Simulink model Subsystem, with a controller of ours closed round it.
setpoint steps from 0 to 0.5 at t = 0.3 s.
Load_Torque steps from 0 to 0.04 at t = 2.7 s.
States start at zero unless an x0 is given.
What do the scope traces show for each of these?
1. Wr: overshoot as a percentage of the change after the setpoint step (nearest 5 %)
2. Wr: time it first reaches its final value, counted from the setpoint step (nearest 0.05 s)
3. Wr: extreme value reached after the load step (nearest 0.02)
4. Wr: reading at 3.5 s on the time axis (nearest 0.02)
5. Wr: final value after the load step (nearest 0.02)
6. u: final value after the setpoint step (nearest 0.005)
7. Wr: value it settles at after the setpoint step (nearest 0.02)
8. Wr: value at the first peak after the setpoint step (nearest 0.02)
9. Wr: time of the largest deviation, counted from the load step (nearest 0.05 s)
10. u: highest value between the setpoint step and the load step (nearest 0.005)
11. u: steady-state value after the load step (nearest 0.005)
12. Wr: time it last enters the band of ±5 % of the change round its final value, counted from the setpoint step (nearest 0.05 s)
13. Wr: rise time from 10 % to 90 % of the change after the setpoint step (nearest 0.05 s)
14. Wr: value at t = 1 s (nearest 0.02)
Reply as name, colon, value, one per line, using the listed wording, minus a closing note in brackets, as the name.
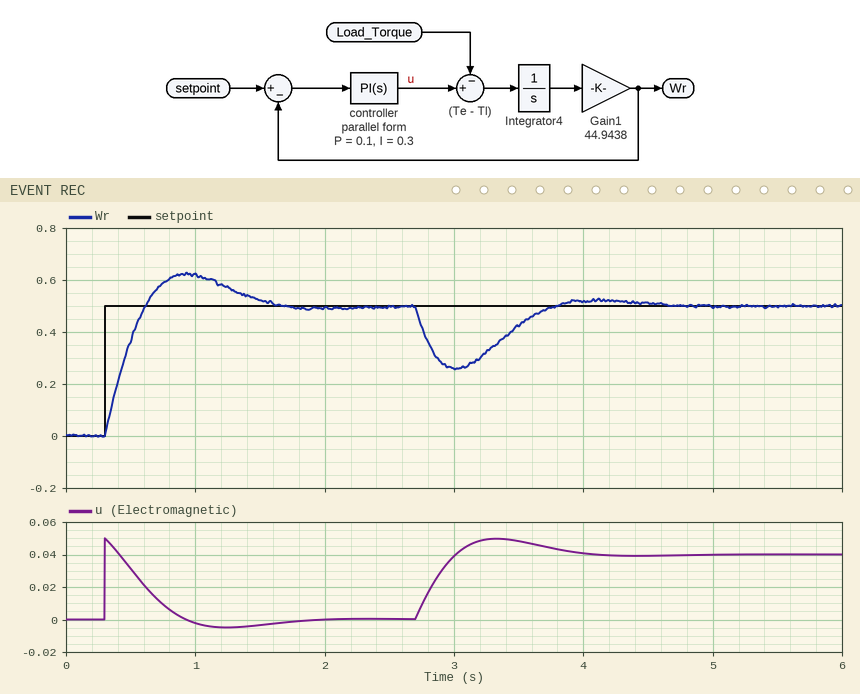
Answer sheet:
Wr: overshoot as a percentage of the change after the setpoint step: 25 %
Wr: time it first reaches its final value, counted from the setpoint step: 0.30 s
Wr: extreme value reached after the load step: 0.26
Wr: reading at 3.5 s on the time axis: 0.42
Wr: final value after the load step: 0.50
u: final value after the setpoint step: 0.000
Wr: value it settles at after the setpoint step: 0.50
Wr: value at the first peak after the setpoint step: 0.62
Wr: time of the largest deviation, counted from the load step: 0.30 s
u: highest value between the setpoint step and the load step: 0.050
u: steady-state value after the load step: 0.040
Wr: time it last enters the band of ±5 % of the change round its final value, counted from the setpoint step: 1.20 s
Wr: rise time from 10 % to 90 % of the change after the setpoint step: 0.25 s
Wr: value at t = 1 s: 0.62
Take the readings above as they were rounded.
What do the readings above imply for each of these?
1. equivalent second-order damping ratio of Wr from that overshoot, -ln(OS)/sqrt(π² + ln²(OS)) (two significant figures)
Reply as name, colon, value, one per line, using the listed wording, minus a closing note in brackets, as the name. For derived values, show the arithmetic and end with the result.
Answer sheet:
equivalent second-order damping ratio of Wr from that overshoot, -ln(OS)/sqrt(π² + ln²(OS)): ln(0.25) = -1.386; 1.386 / sqrt(9.870 + 1.922) = 0.40
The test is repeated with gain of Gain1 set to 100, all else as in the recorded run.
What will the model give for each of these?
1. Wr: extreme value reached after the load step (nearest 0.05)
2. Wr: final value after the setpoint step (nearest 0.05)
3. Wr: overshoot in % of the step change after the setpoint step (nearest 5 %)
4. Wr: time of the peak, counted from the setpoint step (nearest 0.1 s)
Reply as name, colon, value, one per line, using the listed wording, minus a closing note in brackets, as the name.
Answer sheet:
Wr: extreme value reached after the load step: 0.20
Wr: final value after the setpoint step: 0.50
Wr: overshoot in % of the step change after the setpoint step: 15 %
Wr: time of the peak, counted from the setpoint step: 0.4 s
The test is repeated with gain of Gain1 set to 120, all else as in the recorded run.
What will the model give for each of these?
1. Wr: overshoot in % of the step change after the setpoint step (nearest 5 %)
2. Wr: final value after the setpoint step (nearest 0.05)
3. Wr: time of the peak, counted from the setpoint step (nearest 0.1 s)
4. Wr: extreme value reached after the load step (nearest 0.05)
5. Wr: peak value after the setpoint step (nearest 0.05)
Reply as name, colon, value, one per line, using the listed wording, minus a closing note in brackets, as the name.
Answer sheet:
Wr: overshoot in % of the step change after the setpoint step: 15 %
Wr: final value after the setpoint step: 0.50
Wr: time of the peak, counted from the setpoint step: 0.3 s
Wr: extreme value reached after the load step: 0.20
Wr: peak value after the setpoint step: 0.55
